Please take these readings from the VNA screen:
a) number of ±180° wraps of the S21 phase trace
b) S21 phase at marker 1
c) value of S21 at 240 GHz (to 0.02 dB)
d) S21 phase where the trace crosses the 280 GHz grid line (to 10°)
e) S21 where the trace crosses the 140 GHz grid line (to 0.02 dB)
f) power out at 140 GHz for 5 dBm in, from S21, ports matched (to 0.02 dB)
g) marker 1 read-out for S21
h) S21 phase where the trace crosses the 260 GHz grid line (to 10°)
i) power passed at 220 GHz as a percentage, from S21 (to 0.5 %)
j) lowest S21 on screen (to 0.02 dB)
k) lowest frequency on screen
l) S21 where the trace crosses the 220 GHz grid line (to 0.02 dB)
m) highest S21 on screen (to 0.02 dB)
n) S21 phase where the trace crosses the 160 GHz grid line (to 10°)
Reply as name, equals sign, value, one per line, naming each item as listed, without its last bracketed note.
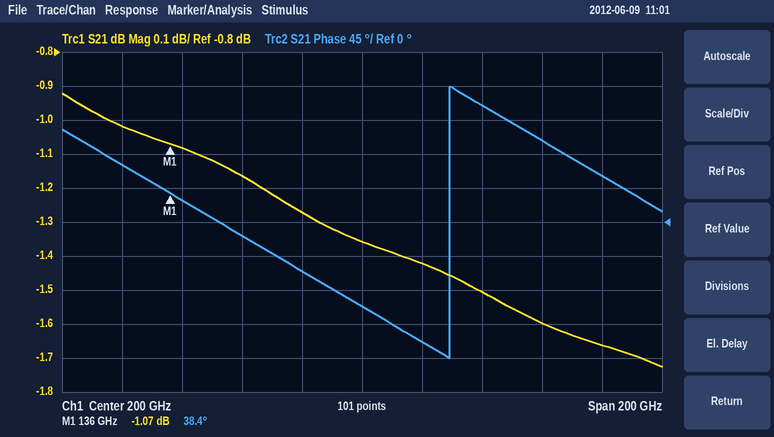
number of ±180° wraps of the S21 phase trace = 1
S21 phase at marker 1 = 38.4°
value of S21 at 240 GHz = -1.50 dB
S21 phase where the trace crosses the 280 GHz grid line = 60°
S21 where the trace crosses the 140 GHz grid line = -1.08 dB
power out at 140 GHz for 5 dBm in, from S21, ports matched = 3.92 dBm
marker 1 read-out for S21 = -1.07 dB
S21 phase where the trace crosses the 260 GHz grid line = 110°
power passed at 220 GHz as a percentage, from S21 = 72.0 %
lowest S21 on screen = -1.72 dB
lowest frequency on screen = 100 GHz
S21 where the trace crosses the 220 GHz grid line = -1.42 dB
highest S21 on screen = -0.92 dB
S21 phase where the trace crosses the 160 GHz grid line = -20°
